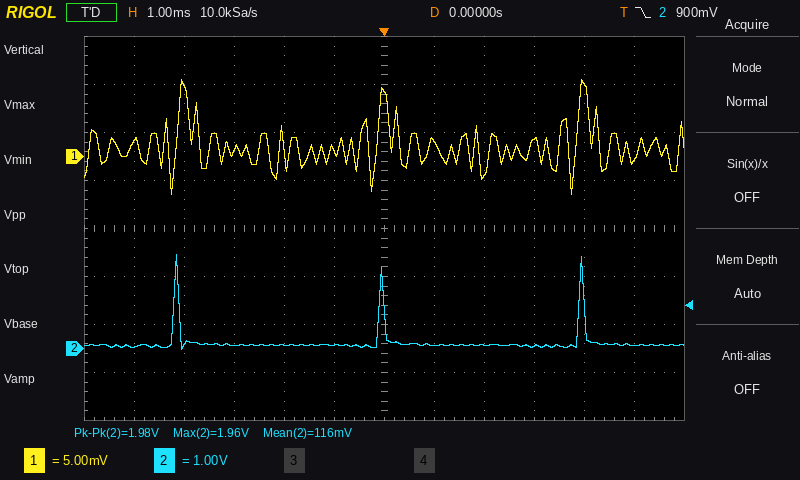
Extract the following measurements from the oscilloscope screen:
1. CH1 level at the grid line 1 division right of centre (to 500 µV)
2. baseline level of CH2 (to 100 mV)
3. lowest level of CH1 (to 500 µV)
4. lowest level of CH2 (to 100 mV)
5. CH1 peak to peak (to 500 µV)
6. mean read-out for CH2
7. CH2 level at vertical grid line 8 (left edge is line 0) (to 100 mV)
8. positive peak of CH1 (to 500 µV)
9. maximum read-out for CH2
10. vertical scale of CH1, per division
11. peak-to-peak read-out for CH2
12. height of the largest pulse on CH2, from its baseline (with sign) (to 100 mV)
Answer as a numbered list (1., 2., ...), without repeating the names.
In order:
1. 1.5 mV
2. 100 mV
3. -4.0 mV
4. 0.0 V
5. 12.0 mV
6. 116 mV
7. 100 mV
8. 8.0 mV
9. 1.96 V
10. 5 mV
11. 1.98 V
12. +1.9 V
